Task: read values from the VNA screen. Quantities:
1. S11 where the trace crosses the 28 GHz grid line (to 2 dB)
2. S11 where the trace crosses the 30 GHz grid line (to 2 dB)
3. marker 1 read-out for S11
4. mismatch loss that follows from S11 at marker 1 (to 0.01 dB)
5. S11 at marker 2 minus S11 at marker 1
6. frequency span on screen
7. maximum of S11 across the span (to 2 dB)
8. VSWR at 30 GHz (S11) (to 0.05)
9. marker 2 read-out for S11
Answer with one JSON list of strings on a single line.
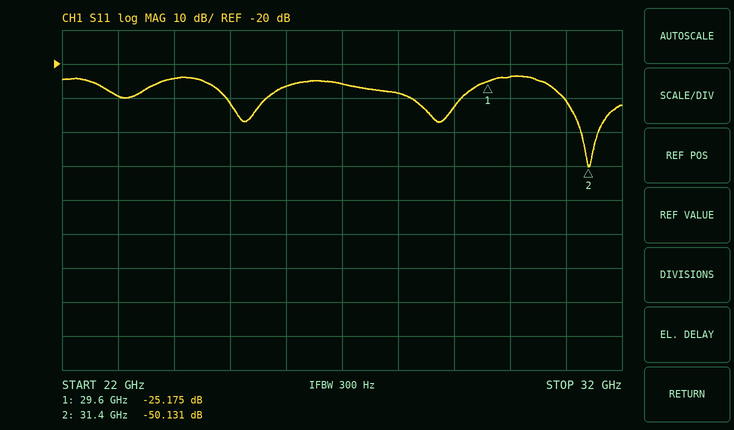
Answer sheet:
["-28 dB", "-24 dB", "-25.175 dB", "0.01 dB", "-24.956 dB", "10 GHz", "-24 dB", "1.15", "-50.131 dB"]
